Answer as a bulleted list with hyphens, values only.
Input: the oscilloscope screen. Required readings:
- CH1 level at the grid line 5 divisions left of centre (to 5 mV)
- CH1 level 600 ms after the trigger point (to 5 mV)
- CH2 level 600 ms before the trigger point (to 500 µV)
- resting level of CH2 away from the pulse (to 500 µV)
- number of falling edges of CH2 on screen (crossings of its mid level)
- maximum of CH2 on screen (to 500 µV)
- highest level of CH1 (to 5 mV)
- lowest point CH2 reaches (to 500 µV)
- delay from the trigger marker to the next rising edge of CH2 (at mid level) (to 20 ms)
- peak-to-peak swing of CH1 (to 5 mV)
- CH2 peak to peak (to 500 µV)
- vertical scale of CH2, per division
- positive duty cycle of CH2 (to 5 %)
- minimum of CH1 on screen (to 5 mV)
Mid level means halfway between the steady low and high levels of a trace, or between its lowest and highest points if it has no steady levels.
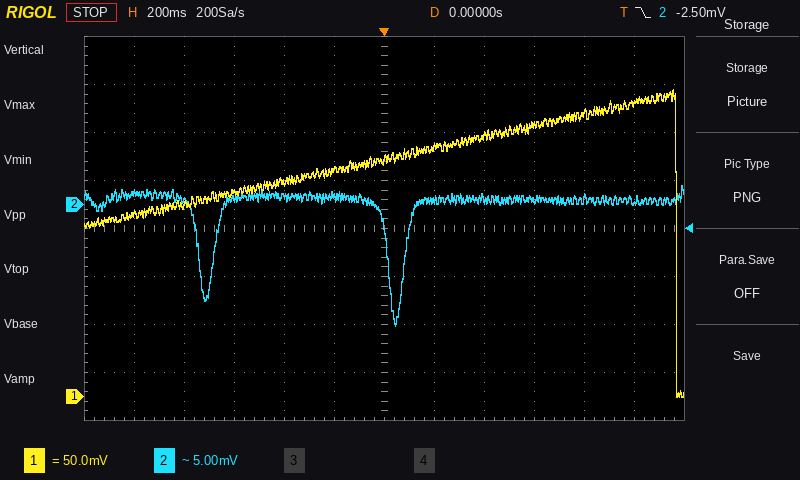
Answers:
- 190 mV
- 285 mV
- 500 µV
- 500 µV
- 2
- 2.0 mV
- 320 mV
- -12.5 mV
- 80 ms
- 320 mV
- 14.5 mV
- 5 mV
- 90 %
- 0 mV
